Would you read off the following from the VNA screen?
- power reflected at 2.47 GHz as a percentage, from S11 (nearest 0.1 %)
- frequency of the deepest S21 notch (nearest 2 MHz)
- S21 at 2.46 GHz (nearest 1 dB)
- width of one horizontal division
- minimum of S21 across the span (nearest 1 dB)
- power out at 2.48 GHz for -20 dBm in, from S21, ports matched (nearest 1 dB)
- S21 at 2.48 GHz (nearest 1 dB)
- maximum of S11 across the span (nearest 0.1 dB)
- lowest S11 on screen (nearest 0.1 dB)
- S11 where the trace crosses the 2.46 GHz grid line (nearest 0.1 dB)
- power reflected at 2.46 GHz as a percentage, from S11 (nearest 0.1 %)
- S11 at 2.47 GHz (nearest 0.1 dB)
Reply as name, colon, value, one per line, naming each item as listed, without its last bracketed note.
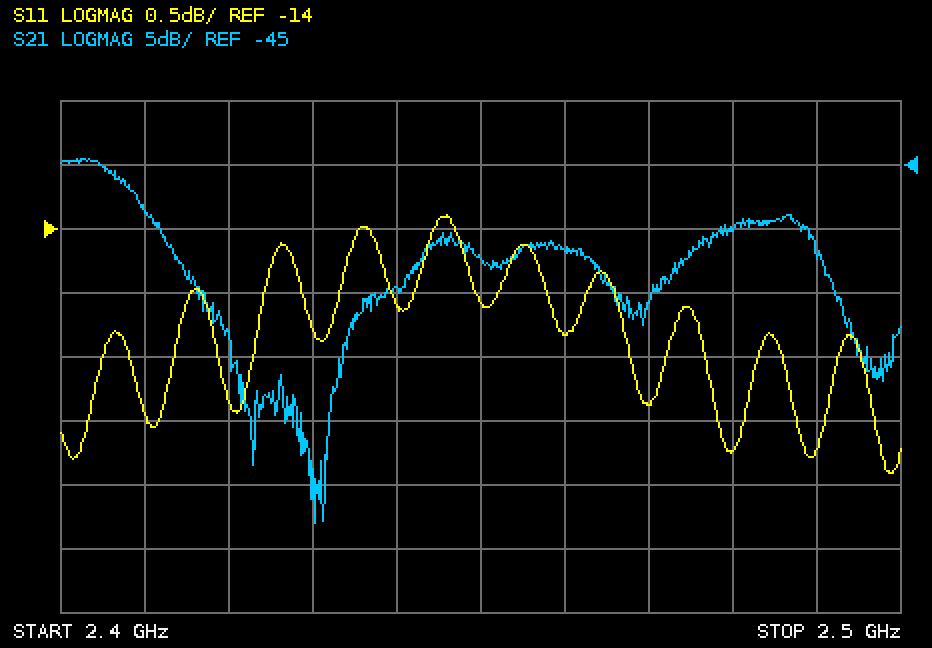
power reflected at 2.47 GHz as a percentage, from S11: 2.9 %
frequency of the deepest S21 notch: 2.430 GHz
S21 at 2.46 GHz: -52 dB
width of one horizontal division: 10 MHz
minimum of S21 across the span: -73 dB
power out at 2.48 GHz for -20 dBm in, from S21, ports matched: -70 dBm
S21 at 2.48 GHz: -50 dB
maximum of S11 across the span: -13.9 dB
lowest S11 on screen: -15.9 dB
S11 where the trace crosses the 2.46 GHz grid line: -14.8 dB
power reflected at 2.46 GHz as a percentage, from S11: 3.3 %
S11 at 2.47 GHz: -15.4 dB
